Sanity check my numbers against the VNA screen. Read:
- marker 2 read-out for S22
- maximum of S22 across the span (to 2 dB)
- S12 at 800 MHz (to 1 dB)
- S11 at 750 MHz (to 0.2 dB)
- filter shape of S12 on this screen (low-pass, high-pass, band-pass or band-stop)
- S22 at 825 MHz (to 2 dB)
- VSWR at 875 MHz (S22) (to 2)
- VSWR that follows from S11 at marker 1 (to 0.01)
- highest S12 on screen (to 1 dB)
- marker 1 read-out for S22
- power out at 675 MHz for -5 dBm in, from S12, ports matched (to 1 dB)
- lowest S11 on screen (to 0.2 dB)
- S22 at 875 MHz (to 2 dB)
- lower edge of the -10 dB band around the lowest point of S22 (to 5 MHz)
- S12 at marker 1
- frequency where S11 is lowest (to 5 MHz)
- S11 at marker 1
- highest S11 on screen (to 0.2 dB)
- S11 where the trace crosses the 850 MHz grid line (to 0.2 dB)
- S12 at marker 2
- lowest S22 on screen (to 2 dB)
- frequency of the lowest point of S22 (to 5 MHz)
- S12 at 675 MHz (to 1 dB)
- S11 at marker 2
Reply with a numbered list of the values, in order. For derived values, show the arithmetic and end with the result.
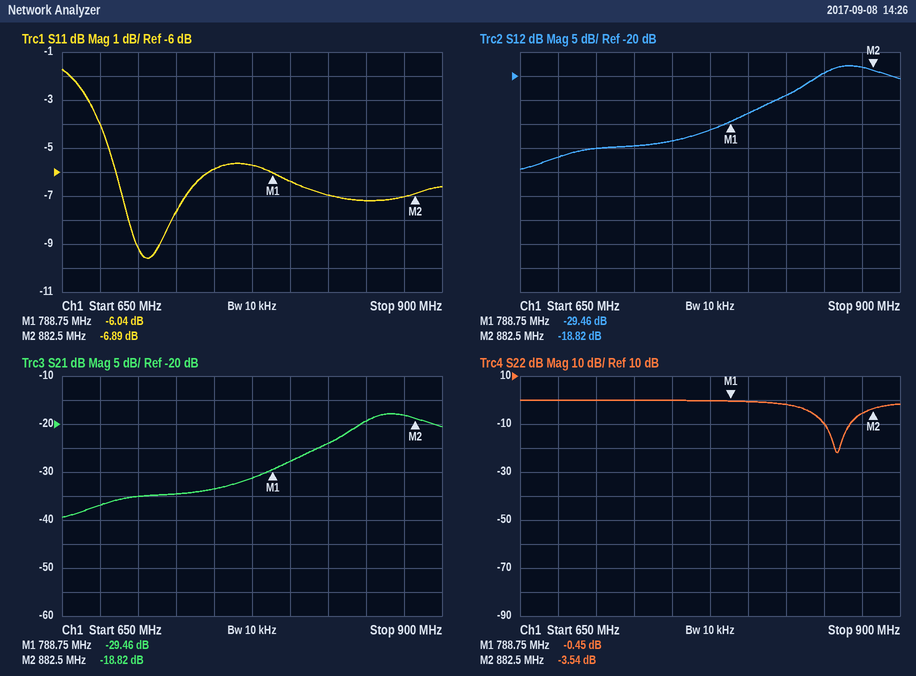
1. -3.54 dB
2. 0 dB
3. -28 dB
4. -5.8 dB
5. high-pass
6. -2 dB
7. |Γ| = 10^(-6/20) = 0.5012; VSWR = (1 + 0.5012)/(1 − 0.5012) ≈ 3.01, so 4 to the nearest 2
8. (1 + 0.4989)/(1 − 0.4989) ≈ 2.99
9. -18 dB
10. -0.45 dB
11. -5 dBm + (-37 dB) = -42 dBm
12. -9.6 dB
13. -6 dB
14. 850 MHz
15. -29.46 dB
16. 705 MHz
17. -6.04 dB
18. -1.8 dB
19. -7.2 dB
20. -18.82 dB
21. -22 dB
22. 860 MHz
23. -37 dB
24. -6.89 dB
